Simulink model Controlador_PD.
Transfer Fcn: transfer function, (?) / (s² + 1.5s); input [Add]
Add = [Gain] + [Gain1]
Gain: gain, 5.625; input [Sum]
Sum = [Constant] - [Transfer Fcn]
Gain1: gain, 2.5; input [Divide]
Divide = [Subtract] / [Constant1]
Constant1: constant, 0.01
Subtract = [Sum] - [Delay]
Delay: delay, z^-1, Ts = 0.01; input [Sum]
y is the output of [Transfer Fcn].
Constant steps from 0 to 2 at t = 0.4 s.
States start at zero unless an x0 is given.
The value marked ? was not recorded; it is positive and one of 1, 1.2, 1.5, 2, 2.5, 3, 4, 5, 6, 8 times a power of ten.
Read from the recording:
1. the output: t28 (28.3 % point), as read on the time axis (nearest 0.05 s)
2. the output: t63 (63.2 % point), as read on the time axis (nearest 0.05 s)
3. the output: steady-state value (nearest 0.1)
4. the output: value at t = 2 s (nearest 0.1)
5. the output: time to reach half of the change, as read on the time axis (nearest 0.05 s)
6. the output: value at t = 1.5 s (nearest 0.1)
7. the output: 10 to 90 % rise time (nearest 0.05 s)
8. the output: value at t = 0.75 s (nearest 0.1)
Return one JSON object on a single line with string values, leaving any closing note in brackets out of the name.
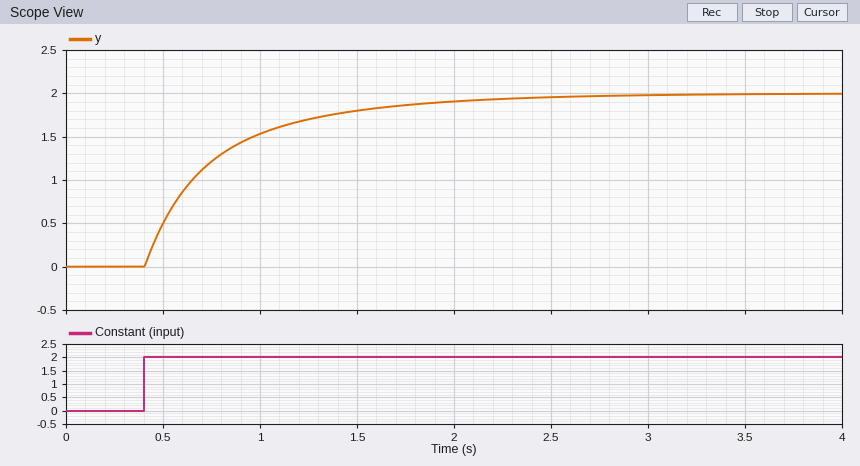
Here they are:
{"the output: t28 (28.3 % point), as read on the time axis": "0.50 s", "the output: t63 (63.2 % point), as read on the time axis": "0.80 s", "the output: steady-state value": "2.0", "the output: value at t = 2 s": "1.9", "the output: time to reach half of the change, as read on the time axis": "0.65 s", "the output: value at t = 1.5 s": "1.8", "the output: 10 to 90 % rise time": "1.05 s", "the output: value at t = 0.75 s": "1.2"}
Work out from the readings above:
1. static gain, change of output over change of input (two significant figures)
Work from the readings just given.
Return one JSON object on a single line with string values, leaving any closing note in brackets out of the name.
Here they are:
{"static gain, change of output over change of input": "1.0"}
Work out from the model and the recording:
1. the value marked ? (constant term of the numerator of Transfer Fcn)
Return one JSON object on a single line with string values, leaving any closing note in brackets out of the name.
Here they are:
{"the value marked ?": "1.2"}
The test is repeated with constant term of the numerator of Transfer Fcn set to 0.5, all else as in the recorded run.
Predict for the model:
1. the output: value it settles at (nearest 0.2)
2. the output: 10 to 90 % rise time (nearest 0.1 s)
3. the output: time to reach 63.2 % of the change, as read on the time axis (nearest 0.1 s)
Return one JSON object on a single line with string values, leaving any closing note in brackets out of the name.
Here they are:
{"the output: value it settles at": "2.0", "the output: 10 to 90 % rise time": "1.6 s", "the output: time to reach 63.2 % of the change, as read on the time axis": "1.2 s"}
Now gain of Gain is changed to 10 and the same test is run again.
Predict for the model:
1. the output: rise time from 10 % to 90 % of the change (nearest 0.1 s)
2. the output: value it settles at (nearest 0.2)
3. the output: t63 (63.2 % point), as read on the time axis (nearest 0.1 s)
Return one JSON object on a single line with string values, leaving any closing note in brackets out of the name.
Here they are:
{"the output: rise time from 10 % to 90 % of the change": "0.5 s", "the output: value it settles at": "2.0", "the output: t63 (63.2 % point), as read on the time axis": "0.7 s"}
